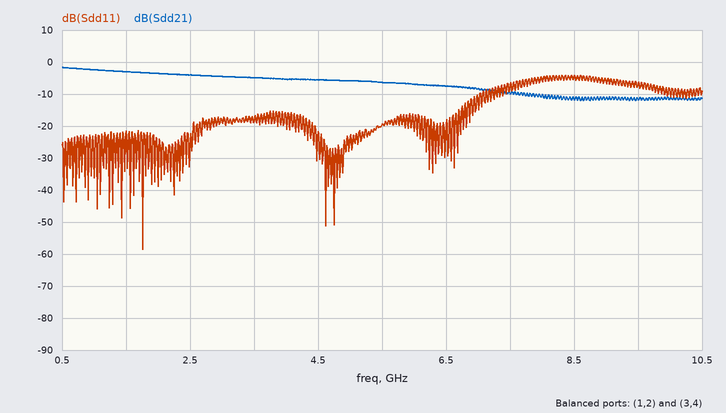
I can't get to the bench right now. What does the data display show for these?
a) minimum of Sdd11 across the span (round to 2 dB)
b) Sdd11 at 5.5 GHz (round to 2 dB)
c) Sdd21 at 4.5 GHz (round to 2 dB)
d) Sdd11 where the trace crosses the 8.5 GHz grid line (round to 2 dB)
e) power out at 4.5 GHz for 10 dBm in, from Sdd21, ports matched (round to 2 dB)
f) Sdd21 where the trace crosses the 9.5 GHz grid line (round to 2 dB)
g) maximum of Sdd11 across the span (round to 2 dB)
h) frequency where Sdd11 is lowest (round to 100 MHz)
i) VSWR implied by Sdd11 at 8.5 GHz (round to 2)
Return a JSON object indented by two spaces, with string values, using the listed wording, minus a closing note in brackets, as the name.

{
  "minimum of Sdd11 across the span": "-58 dB",
  "Sdd11 at 5.5 GHz": "-20 dB",
  "Sdd21 at 4.5 GHz": "-6 dB",
  "Sdd11 where the trace crosses the 8.5 GHz grid line": "-4 dB",
  "power out at 4.5 GHz for 10 dBm in, from Sdd21, ports matched": "4 dBm",
  "Sdd21 where the trace crosses the 9.5 GHz grid line": "-12 dB",
  "maximum of Sdd11 across the span": "-4 dB",
  "frequency where Sdd11 is lowest": "1.8 GHz",
  "VSWR implied by Sdd11 at 8.5 GHz": "4"
}
